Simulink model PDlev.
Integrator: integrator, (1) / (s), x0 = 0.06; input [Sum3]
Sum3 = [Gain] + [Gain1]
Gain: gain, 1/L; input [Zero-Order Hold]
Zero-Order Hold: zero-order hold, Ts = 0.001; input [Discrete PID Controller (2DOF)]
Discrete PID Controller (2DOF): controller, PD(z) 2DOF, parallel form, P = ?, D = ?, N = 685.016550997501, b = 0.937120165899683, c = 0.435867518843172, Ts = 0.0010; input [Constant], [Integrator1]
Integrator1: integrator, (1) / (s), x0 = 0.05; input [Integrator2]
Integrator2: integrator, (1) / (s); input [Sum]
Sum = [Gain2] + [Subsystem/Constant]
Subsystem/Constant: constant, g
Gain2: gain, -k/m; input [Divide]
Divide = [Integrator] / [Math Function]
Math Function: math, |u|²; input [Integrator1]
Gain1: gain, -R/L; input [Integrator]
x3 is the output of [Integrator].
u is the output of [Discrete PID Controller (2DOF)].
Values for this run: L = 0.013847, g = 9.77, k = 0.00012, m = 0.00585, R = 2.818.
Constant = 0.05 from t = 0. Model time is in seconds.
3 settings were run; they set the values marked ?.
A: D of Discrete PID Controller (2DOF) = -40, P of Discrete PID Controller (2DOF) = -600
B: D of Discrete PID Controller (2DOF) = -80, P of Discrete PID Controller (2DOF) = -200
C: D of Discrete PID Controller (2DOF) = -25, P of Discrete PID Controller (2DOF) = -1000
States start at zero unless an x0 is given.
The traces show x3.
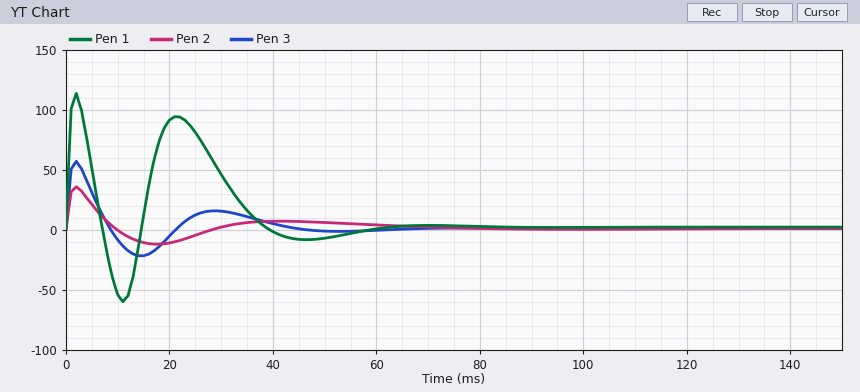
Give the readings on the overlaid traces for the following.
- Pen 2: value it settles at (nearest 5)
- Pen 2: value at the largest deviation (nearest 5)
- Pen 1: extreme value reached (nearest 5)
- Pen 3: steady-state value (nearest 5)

0
35
115
0
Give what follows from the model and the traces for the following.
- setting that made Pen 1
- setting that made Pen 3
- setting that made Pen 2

B
A
C
